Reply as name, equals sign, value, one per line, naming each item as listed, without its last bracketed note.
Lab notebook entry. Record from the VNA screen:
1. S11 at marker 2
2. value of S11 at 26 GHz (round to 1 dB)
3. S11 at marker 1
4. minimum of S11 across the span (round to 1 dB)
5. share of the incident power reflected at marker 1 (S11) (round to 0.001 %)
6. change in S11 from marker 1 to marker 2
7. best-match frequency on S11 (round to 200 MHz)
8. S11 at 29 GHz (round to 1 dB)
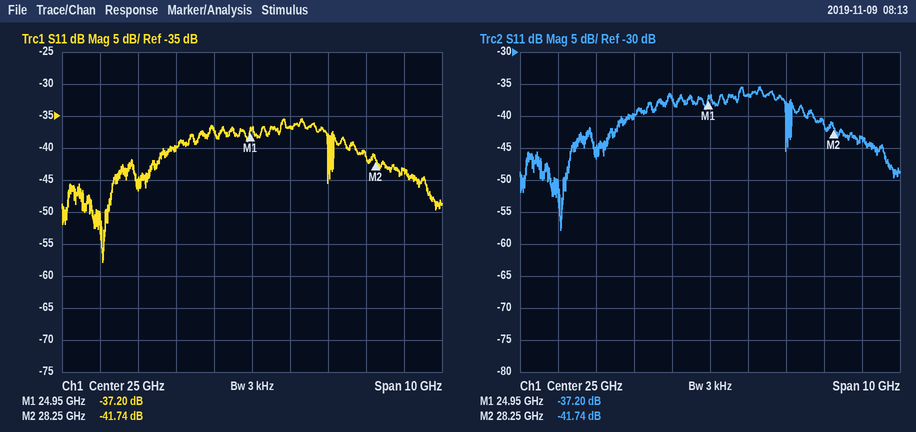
S11 at marker 2 = -41.74 dB
value of S11 at 26 GHz = -37 dB
S11 at marker 1 = -37.20 dB
minimum of S11 across the span = -58 dB
share of the incident power reflected at marker 1 (S11) = 0.019 %
change in S11 from marker 1 to marker 2 = -4.54 dB
best-match frequency on S11 = 21.0 GHz
S11 at 29 GHz = -43 dB
